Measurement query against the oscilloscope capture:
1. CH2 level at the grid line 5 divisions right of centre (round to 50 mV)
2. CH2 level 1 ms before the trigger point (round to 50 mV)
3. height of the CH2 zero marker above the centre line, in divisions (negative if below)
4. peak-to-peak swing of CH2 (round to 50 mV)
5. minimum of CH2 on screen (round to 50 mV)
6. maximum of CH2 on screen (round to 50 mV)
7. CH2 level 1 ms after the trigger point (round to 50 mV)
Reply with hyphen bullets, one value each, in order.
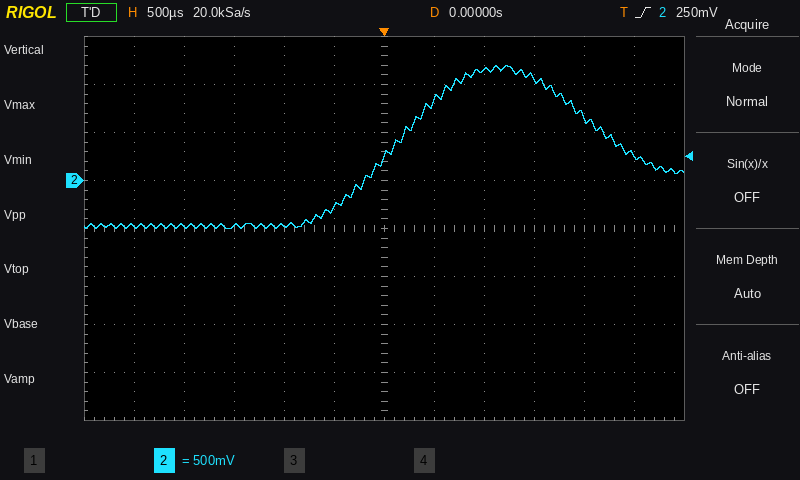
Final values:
- 250 mV
- -450 mV
- +1.0 div
- 1.70 V
- -500 mV
- 1.20 V
- 1.15 V
